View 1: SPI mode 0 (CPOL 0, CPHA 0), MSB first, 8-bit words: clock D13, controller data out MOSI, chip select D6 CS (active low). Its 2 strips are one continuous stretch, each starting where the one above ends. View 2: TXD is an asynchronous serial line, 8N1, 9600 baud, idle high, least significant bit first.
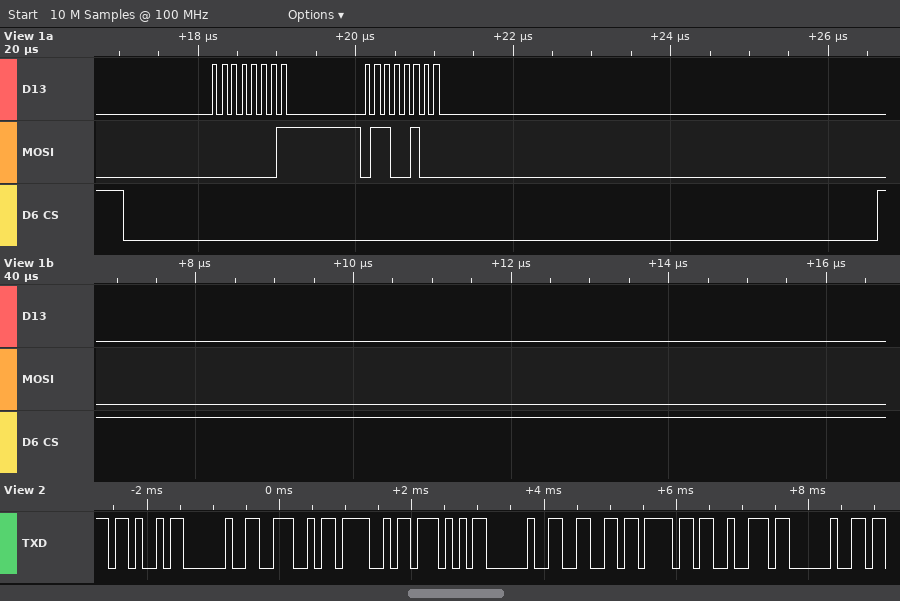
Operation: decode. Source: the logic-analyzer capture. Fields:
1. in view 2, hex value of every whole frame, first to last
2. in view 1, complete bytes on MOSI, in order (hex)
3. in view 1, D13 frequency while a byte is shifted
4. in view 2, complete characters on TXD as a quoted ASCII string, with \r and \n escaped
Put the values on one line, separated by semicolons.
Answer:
4B 20 4E 4F 57 20 66 6F 72 20; 01 64; 8 MHz; "K NOW for "
